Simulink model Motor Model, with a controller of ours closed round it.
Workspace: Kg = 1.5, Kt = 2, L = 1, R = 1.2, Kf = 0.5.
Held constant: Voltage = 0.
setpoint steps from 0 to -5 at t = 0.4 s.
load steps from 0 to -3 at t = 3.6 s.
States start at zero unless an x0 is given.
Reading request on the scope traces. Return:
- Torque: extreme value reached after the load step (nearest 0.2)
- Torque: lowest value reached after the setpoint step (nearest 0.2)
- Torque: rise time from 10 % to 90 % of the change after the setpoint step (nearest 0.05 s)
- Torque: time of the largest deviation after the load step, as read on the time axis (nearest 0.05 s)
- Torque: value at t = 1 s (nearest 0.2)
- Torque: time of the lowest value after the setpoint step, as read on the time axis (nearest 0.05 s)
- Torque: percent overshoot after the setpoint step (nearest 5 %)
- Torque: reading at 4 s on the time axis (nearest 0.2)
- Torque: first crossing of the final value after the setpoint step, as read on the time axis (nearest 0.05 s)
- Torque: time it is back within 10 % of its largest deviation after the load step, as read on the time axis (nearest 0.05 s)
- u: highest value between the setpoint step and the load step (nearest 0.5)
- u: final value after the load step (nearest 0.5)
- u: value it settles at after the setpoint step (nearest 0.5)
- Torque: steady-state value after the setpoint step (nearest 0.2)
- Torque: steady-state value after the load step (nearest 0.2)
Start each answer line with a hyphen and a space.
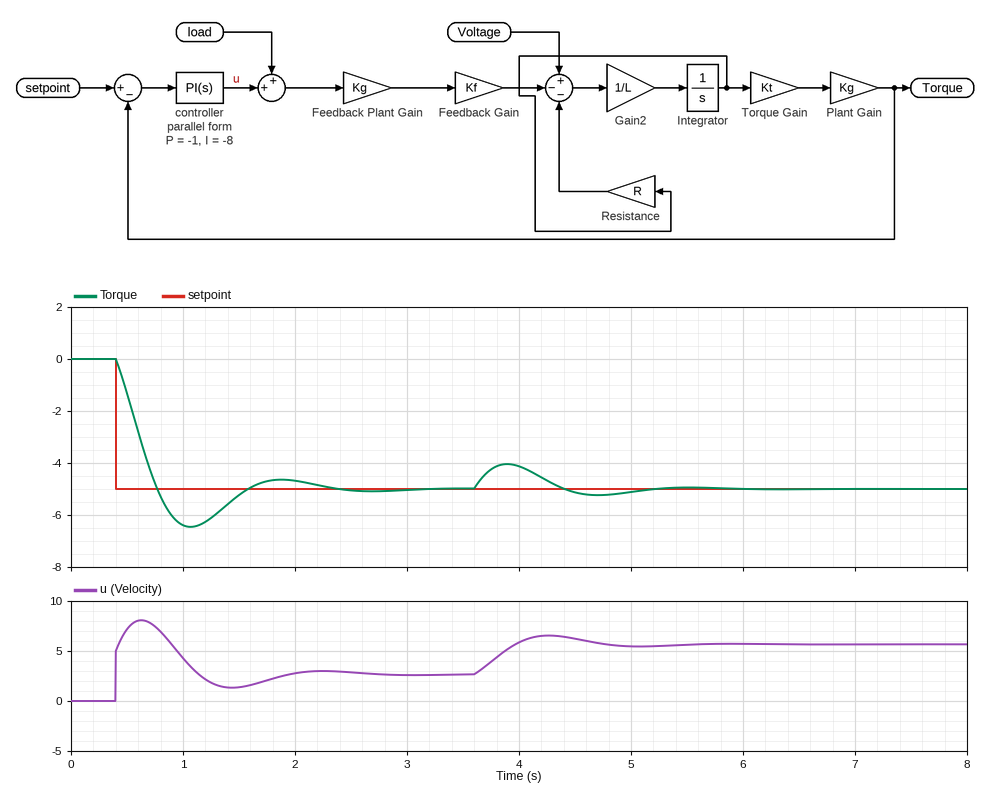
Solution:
- -4.0
- -6.4
- 0.30 s
- 3.90 s
- -6.4
- 1.05 s
- 30 %
- -4.2
- 0.75 s
- 5.05 s
- 8.0
- 5.5
- 2.5
- -5.0
- -5.0
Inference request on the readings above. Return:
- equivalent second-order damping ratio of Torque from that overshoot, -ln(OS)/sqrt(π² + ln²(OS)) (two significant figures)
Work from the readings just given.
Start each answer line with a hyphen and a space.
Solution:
- 0.36
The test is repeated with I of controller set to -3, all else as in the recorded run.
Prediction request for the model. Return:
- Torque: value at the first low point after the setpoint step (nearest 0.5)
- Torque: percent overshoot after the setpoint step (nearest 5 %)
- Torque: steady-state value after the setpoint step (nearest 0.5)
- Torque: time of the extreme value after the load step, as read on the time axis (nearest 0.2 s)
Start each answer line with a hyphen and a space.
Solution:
- -5.5
- 10 %
- -5.0
- 4.0 s
